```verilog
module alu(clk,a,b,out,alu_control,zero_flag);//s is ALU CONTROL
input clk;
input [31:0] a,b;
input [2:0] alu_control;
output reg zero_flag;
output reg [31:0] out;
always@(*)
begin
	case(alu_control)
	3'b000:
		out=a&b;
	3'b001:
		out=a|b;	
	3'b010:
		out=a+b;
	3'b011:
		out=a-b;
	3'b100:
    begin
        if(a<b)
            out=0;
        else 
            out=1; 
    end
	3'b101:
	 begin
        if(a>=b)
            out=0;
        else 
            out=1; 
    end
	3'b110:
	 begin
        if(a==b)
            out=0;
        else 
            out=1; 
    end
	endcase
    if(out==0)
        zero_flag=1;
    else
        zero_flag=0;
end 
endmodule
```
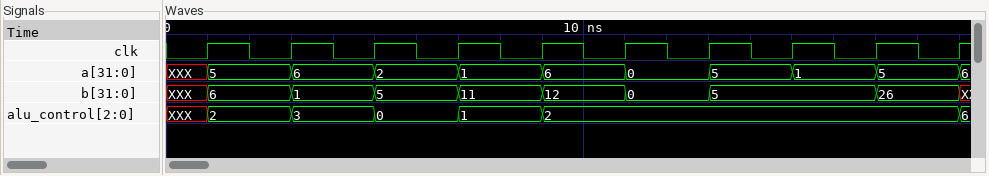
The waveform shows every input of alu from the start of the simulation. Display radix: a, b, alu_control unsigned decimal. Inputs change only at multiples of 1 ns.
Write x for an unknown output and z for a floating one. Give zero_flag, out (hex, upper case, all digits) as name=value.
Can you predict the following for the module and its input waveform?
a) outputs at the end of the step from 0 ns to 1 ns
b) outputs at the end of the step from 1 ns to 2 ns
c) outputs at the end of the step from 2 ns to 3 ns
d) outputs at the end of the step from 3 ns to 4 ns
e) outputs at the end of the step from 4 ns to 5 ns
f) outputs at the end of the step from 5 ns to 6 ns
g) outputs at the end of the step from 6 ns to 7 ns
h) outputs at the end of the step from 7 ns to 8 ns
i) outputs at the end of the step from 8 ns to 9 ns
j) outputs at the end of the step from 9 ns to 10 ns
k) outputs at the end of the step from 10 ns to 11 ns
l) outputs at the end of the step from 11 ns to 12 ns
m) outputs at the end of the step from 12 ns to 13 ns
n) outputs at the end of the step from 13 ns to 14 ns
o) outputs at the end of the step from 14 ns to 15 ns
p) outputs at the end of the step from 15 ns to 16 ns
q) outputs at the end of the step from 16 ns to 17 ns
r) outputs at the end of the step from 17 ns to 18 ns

zero_flag=x, out=x
zero_flag=0, out=0000000B
zero_flag=0, out=0000000B
zero_flag=0, out=00000005
zero_flag=0, out=00000005
zero_flag=1, out=00000000
zero_flag=1, out=00000000
zero_flag=0, out=0000000B
zero_flag=0, out=0000000B
zero_flag=0, out=00000012
zero_flag=0, out=00000012
zero_flag=1, out=00000000
zero_flag=1, out=00000000
zero_flag=0, out=0000000A
zero_flag=0, out=0000000A
zero_flag=0, out=00000006
zero_flag=0, out=00000006
zero_flag=0, out=0000001F
